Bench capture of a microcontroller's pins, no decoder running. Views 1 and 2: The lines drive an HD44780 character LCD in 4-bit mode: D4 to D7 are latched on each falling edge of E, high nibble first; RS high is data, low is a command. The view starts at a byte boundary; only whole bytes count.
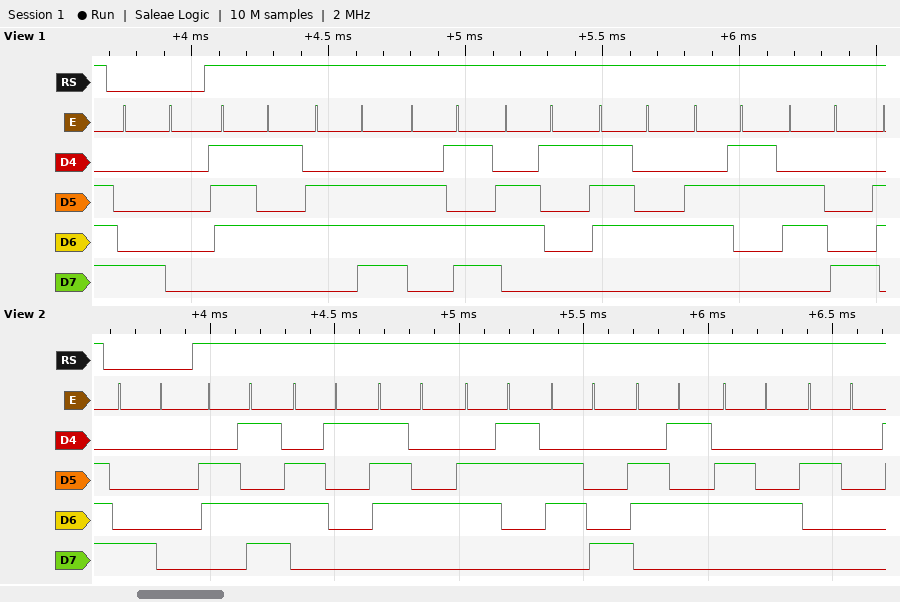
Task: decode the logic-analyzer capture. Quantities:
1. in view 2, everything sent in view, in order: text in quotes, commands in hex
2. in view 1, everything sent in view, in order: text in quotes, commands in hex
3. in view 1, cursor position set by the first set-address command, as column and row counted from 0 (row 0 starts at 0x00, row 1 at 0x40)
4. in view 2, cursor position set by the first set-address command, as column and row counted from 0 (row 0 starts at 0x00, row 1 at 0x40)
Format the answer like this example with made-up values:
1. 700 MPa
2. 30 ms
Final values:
1. 0x80 "matched "
2. 0x80 "unmatch"
3. column 0, row 0
4. column 0, row 0
